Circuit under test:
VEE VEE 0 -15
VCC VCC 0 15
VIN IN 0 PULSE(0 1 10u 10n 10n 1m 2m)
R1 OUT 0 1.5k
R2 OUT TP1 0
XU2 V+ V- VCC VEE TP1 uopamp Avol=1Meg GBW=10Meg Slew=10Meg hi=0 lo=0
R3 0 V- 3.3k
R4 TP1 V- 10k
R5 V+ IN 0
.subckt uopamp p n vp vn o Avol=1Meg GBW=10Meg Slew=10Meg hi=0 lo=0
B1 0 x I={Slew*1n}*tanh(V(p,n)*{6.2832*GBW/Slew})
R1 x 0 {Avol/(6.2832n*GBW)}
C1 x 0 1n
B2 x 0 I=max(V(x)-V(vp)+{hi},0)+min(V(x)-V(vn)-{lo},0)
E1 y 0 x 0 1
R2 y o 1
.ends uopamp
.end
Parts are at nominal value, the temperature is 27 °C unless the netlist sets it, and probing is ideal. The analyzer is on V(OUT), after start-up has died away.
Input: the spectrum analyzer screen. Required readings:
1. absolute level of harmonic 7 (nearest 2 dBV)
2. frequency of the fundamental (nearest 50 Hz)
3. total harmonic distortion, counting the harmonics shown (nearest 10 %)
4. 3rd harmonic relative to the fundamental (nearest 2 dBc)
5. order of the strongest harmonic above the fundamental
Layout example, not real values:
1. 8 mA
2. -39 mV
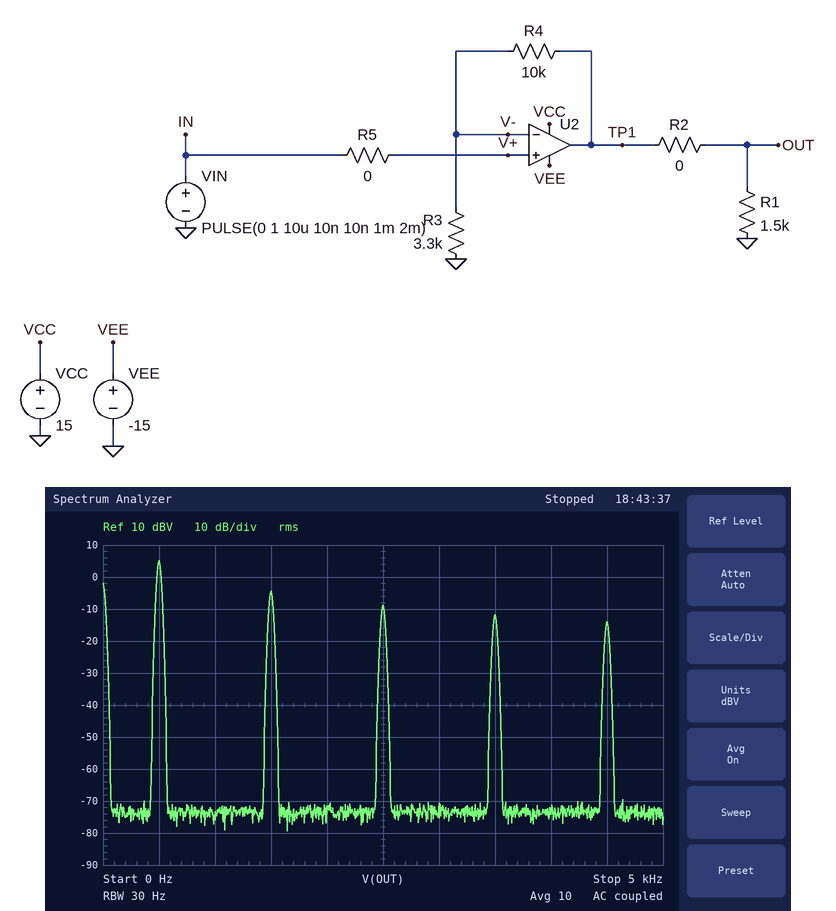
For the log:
1. -12 dBV
2. 500 Hz
3. 40 %
4. -10 dBc
5. 3
